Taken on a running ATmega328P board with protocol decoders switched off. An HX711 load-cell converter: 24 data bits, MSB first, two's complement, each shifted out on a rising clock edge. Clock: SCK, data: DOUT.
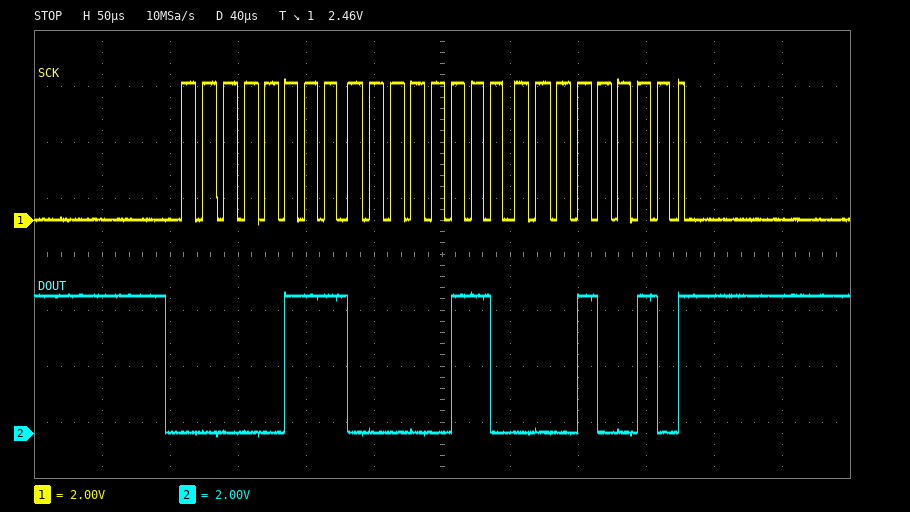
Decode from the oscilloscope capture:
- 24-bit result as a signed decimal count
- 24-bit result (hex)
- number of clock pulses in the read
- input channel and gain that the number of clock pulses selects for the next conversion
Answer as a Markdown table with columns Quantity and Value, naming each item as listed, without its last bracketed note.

| Quantity | Value |
|---|---|
| 24-bit result as a signed decimal count | 460306 |
| 24-bit result | 0x070612 |
| number of clock pulses in the read | 25 |
| input channel and gain that the number of clock pulses selects for the next conversion | channel A, gain 128 |
